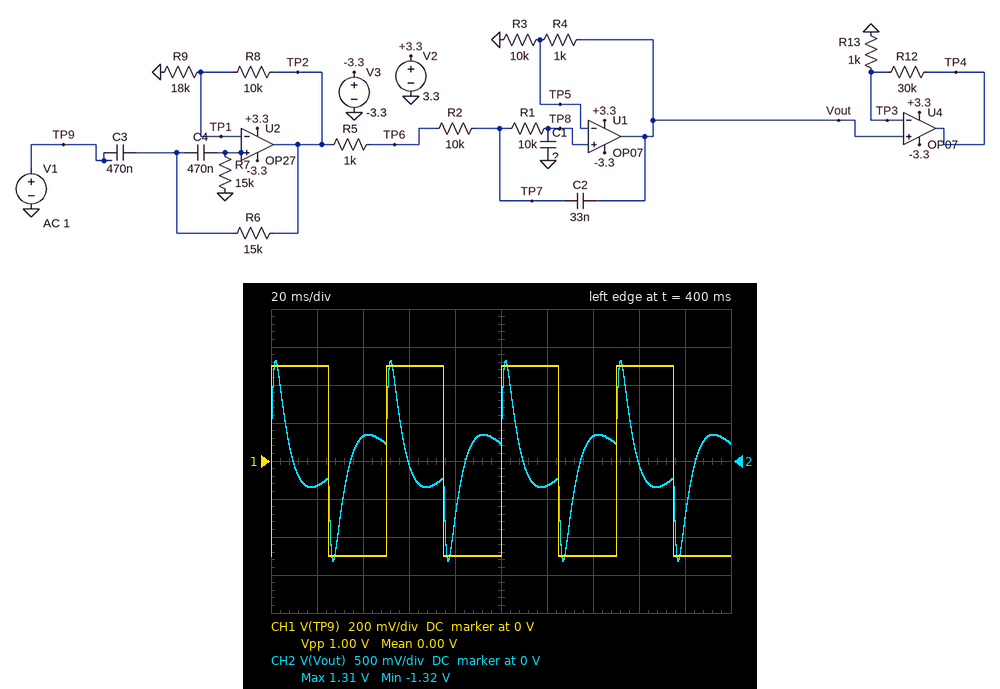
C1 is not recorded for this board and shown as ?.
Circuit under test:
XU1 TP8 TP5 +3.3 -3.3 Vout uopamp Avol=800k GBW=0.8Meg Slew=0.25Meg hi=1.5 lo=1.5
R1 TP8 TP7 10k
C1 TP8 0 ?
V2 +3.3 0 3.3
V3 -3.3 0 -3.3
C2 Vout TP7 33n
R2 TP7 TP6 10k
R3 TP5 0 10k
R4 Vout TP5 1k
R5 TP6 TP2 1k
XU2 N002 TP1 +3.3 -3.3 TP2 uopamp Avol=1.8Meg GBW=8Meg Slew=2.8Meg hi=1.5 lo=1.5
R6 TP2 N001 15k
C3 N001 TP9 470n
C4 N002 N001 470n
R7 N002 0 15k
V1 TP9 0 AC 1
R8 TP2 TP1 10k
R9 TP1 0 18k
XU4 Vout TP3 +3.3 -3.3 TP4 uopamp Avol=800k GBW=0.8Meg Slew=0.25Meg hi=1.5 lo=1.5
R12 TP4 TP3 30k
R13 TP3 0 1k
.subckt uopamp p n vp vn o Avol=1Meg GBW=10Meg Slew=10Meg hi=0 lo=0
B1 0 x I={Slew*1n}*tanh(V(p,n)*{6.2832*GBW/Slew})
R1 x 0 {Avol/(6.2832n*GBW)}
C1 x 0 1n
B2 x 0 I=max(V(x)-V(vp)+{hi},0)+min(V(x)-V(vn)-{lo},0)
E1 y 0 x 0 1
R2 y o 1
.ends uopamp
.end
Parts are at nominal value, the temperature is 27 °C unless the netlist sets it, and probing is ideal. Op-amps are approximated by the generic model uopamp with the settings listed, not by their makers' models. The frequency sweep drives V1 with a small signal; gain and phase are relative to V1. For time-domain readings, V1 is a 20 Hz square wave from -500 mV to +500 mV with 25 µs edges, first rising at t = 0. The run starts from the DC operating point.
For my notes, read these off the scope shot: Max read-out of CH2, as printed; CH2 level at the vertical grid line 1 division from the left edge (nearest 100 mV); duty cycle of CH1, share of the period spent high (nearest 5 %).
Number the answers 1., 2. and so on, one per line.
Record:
1. 1.31 V
2. -300 mV
3. 50 %
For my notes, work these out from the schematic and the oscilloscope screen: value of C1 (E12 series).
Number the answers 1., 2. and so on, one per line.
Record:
1. 56 nF
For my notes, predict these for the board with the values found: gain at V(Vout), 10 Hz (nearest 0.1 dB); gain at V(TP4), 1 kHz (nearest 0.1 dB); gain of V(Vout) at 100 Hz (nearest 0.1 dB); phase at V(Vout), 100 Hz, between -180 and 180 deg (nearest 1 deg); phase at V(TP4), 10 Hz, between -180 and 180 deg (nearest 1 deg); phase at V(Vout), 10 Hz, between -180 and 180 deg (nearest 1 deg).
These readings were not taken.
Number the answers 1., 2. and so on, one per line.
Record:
1. -9.7 dB
2. 14.5 dB
3. 3.3 dB
4. -19 deg
5. 137 deg
6. 137 deg
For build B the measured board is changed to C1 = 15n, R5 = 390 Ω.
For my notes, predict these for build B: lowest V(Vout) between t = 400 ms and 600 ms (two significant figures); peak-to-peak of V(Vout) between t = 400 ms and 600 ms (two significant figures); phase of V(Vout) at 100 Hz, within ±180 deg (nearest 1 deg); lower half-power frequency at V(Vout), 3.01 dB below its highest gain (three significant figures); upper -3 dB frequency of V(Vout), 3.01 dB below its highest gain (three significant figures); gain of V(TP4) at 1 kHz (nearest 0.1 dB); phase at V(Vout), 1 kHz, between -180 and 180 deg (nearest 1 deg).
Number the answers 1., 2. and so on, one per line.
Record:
1. -1.8 V
2. 3.6 V
3. 9 deg
4. 24.1 Hz
5. 782 Hz
6. 28.5 dB
7. -119 deg
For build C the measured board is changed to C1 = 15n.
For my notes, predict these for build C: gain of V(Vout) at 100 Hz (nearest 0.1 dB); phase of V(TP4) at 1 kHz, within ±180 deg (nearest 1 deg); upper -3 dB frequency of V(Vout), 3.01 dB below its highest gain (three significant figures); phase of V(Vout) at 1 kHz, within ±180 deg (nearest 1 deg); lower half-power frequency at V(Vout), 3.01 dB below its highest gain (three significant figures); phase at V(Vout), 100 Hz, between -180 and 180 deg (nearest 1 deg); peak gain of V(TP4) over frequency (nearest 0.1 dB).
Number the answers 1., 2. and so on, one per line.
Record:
1. 4.7 dB
2. -124 deg
3. 761 Hz
4. -122 deg
5. 24.2 Hz
6. 9 deg
7. 34.9 dB
